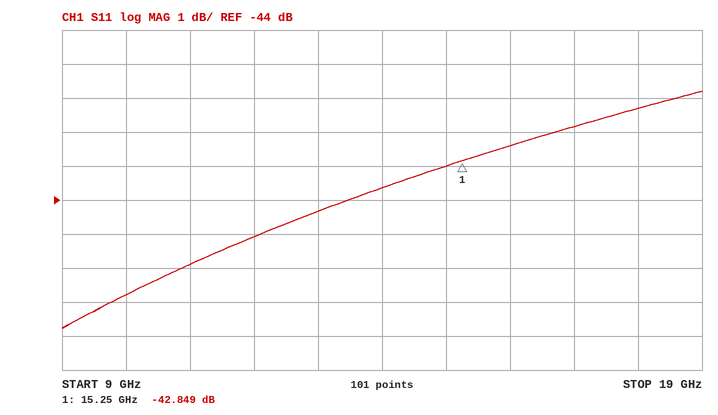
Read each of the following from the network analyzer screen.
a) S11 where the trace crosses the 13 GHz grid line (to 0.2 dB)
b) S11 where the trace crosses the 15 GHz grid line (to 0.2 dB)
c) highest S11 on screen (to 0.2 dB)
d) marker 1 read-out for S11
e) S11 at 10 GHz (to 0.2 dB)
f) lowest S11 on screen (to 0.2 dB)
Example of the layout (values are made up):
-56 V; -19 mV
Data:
-44.4 dB; -43.0 dB; -40.8 dB; -42.849 dB; -46.8 dB; -47.8 dB
